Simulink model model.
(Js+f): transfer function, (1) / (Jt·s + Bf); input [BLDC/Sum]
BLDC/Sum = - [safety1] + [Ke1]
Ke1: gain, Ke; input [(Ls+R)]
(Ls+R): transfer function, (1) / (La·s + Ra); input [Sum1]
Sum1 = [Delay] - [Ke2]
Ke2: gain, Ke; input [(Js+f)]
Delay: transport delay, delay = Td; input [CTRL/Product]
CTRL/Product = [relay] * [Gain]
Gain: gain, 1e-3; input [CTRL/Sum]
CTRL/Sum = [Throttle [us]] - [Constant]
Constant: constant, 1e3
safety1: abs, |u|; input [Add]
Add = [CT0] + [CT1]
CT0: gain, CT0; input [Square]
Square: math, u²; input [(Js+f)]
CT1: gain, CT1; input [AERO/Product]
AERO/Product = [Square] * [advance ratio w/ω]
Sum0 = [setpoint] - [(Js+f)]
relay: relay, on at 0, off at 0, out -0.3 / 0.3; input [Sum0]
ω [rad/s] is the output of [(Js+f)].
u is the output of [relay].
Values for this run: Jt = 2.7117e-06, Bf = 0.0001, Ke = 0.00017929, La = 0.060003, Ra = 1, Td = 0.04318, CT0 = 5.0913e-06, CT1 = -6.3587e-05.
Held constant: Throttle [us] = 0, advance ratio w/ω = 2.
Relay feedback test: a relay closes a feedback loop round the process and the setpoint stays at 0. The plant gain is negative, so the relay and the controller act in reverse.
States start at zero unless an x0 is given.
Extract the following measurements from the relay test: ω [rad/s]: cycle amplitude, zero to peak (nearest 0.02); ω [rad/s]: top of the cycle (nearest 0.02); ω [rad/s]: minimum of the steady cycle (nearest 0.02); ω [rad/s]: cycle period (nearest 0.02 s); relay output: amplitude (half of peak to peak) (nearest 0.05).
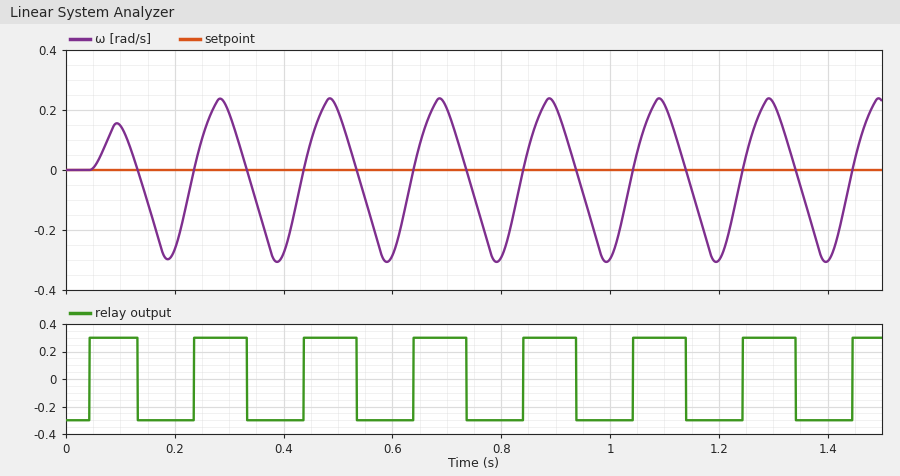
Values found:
0.28
0.24
-0.30
0.20 s
0.30
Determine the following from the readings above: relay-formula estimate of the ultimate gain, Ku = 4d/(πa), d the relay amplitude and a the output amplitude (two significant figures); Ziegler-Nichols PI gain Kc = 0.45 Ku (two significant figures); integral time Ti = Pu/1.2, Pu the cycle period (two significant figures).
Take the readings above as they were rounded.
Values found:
1.4
0.63
0.17 s
